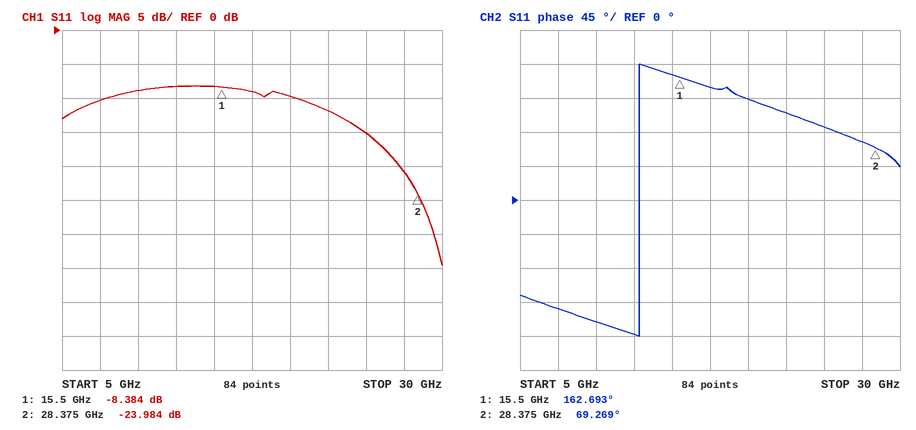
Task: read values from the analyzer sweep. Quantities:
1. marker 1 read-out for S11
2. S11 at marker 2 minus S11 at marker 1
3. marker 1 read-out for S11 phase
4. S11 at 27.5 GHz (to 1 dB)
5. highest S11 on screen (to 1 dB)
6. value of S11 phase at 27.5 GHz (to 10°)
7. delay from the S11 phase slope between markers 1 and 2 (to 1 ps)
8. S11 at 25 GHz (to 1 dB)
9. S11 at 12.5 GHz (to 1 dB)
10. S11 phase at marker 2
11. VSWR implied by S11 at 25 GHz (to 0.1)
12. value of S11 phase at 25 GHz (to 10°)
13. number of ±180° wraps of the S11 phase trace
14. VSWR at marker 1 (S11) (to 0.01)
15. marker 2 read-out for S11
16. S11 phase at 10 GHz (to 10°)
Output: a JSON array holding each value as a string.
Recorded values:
["-8.384 dB", "-15.600 dB", "162.693°", "-21 dB", "-8 dB", "80°", "20 ps", "-15 dB", "-8 dB", "69.269°", "1.4", "100°", "1", "2.23", "-23.984 dB", "-160°"]
